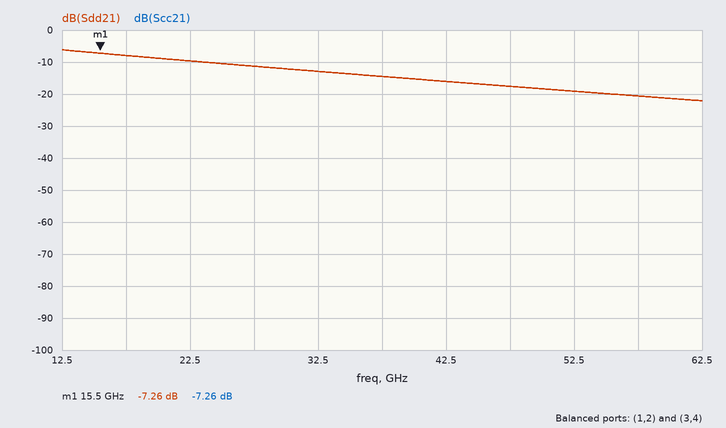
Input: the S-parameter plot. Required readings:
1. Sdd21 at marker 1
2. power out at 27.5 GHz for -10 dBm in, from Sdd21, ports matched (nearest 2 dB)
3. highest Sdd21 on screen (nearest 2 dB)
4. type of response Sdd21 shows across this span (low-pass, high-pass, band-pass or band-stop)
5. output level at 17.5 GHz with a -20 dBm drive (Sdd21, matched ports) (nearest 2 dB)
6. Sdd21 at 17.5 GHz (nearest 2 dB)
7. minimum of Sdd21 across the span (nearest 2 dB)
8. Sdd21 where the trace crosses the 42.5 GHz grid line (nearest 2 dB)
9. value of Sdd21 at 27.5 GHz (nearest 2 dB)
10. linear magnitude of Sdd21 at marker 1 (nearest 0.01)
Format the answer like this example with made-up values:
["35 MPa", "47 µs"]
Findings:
["-7.26 dB", "-22 dBm", "-6 dB", "low-pass", "-28 dBm", "-8 dB", "-22 dB", "-16 dB", "-12 dB", "0.43"]
